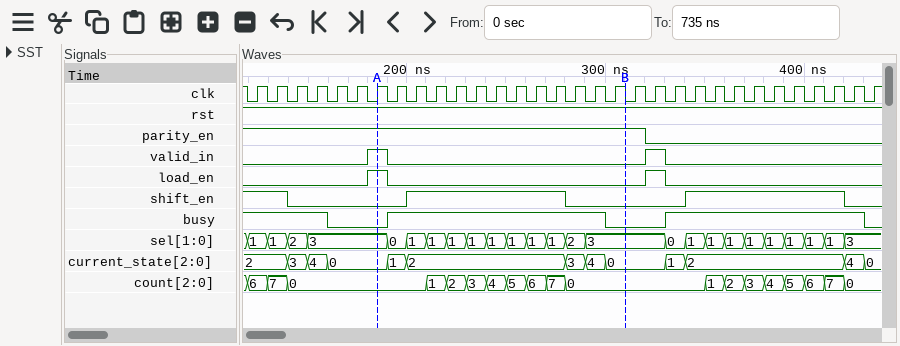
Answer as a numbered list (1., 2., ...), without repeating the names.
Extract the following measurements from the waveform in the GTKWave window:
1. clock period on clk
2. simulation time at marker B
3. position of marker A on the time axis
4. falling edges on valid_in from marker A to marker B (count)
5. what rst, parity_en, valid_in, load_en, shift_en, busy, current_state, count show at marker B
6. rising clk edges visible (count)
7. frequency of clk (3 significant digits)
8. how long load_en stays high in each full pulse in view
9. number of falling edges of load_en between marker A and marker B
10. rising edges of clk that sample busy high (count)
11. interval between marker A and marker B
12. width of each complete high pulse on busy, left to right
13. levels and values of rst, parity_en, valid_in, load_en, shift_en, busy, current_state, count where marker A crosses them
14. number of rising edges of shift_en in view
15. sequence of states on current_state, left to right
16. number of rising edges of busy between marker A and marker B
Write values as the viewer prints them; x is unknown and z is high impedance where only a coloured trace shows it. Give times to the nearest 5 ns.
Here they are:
1. 10 ns
2. 310 ns
3. 185 ns
4. 1
5. rst=1, parity_en=1, valid_in=0, load_en=0, shift_en=0, busy=0, current_state=0, count=0
6. 32
7. 100 MHz
8. 10 ns, 10 ns
9. 1
10. 25
11. 125 ns
12. 110 ns, 100 ns
13. rst=1, parity_en=1, valid_in=1, load_en=1, shift_en=0, busy=0, current_state=0, count=0
14. 2
15. 2, 3, 4, 0, 1, 2, 3, 4, 0, 1, 2, 4, 0
16. 1
